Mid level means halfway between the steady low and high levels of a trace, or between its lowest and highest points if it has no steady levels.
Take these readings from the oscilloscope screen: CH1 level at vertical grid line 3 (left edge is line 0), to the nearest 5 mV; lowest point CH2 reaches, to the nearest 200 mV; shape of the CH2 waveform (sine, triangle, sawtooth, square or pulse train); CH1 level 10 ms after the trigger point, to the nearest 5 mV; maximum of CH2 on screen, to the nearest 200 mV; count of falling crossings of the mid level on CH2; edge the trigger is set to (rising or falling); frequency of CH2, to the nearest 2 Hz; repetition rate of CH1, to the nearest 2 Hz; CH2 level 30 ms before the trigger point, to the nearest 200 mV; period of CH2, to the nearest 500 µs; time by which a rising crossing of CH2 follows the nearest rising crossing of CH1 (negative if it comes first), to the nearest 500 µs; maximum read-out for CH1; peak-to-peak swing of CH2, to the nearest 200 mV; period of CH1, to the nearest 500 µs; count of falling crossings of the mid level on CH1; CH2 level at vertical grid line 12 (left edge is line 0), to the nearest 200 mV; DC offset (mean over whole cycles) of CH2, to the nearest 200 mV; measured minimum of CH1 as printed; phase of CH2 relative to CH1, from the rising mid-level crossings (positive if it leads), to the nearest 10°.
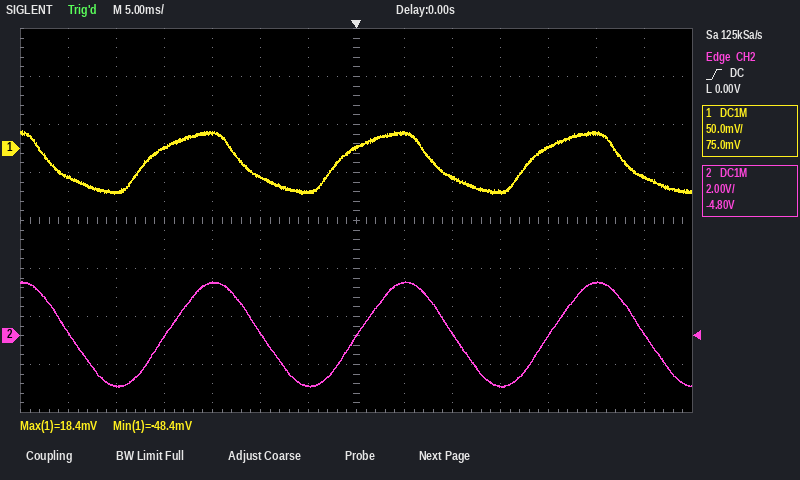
0 mV
-2.2 V
sine
-30 mV
2.2 V
4
rising
50 Hz
50 Hz
200 mV
20.0 ms
+2.0 ms
18.4 mV
4.4 V
20.0 ms
4
2.2 V
0.0 V
-48.4 mV
-40°
